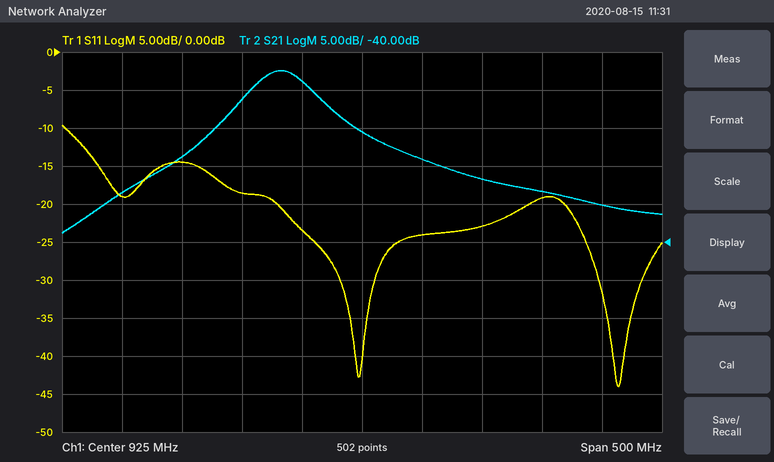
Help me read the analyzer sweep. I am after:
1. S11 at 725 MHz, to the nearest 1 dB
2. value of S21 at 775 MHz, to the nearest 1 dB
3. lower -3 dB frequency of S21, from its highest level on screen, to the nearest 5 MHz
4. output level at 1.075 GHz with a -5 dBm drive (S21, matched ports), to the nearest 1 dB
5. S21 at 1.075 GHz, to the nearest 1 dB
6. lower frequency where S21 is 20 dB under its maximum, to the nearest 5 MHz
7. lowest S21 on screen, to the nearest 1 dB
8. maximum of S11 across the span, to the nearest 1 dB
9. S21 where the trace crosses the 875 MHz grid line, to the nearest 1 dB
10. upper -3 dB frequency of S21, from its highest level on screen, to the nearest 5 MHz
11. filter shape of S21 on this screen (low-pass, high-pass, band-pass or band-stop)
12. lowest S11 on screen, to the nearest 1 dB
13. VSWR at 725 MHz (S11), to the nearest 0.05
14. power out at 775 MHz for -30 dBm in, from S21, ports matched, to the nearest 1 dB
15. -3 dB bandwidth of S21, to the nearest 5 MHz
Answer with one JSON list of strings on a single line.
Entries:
["-19 dB", "-29 dB", "830 MHz", "-38 dBm", "-33 dB", "690 MHz", "-39 dB", "-10 dB", "-19 dB", "885 MHz", "band-pass", "-44 dB", "1.25", "-59 dBm", "55 MHz"]
